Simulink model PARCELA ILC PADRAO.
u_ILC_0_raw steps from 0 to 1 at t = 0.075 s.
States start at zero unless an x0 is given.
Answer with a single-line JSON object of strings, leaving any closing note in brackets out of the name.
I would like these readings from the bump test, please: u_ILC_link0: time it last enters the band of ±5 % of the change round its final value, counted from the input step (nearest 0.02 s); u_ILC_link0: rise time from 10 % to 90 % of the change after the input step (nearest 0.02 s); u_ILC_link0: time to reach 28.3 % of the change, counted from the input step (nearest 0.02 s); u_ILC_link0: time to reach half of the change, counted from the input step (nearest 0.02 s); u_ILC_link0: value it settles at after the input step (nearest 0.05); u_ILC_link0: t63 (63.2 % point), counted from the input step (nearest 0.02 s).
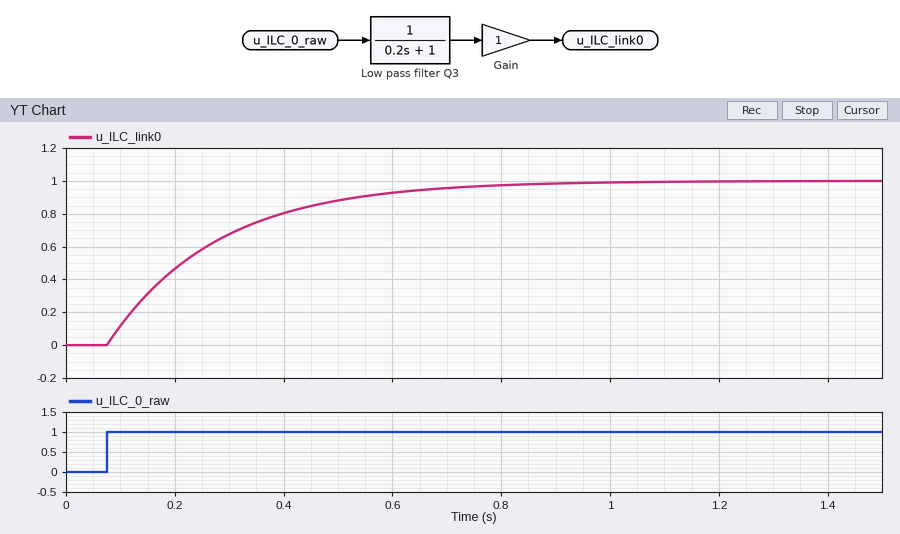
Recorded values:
{"u_ILC_link0: time it last enters the band of ±5 % of the change round its final value, counted from the input step": "0.60 s", "u_ILC_link0: rise time from 10 % to 90 % of the change after the input step": "0.44 s", "u_ILC_link0: time to reach 28.3 % of the change, counted from the input step": "0.06 s", "u_ILC_link0: time to reach half of the change, counted from the input step": "0.14 s", "u_ILC_link0: value it settles at after the input step": "1.00", "u_ILC_link0: t63 (63.2 % point), counted from the input step": "0.20 s"}
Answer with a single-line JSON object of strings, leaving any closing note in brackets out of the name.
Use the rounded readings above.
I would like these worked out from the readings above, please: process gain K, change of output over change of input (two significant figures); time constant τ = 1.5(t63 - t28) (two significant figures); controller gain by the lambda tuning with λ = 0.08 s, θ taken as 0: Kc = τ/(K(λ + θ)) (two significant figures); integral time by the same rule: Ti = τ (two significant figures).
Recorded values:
{"process gain K, change of output over change of input": "1.0", "time constant τ = 1.5(t63 - t28)": "0.21 s", "controller gain by the lambda tuning with λ = 0.08 s, θ taken as 0: Kc = τ/(K(λ + θ))": "2.6", "integral time by the same rule: Ti = τ": "0.21 s"}
